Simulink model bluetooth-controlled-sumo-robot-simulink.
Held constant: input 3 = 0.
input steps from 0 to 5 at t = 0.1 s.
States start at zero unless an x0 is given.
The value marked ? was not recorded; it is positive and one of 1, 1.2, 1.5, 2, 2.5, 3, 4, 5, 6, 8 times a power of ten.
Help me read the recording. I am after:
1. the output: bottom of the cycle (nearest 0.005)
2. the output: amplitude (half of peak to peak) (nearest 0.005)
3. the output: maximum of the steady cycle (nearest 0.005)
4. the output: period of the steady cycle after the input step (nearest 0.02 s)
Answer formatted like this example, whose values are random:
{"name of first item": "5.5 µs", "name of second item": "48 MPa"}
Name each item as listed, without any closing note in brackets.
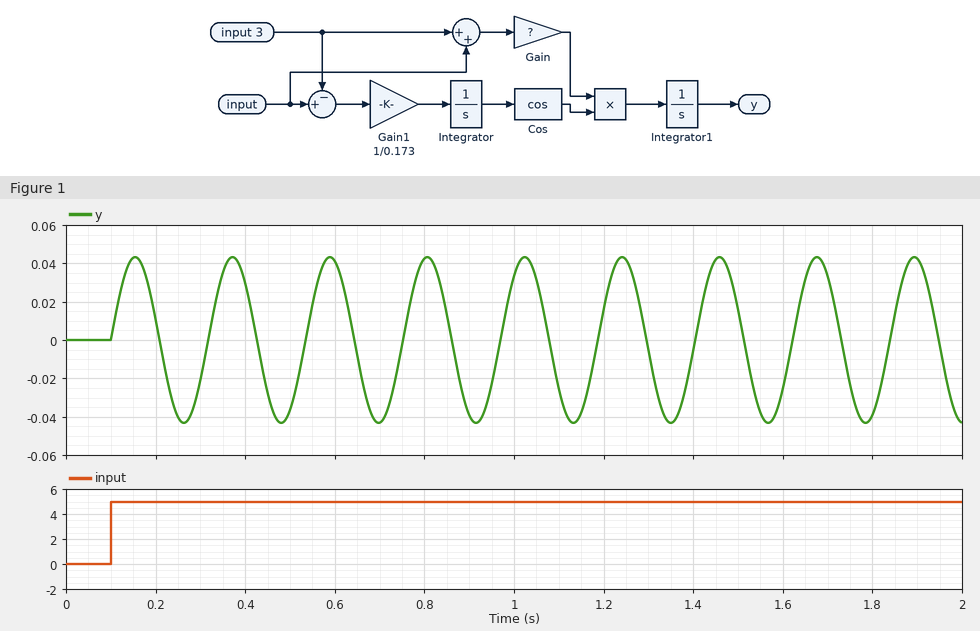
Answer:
{"the output: bottom of the cycle": "-0.045", "the output: amplitude (half of peak to peak)": "0.045", "the output: maximum of the steady cycle": "0.045", "the output: period of the steady cycle after the input step": "0.22 s"}
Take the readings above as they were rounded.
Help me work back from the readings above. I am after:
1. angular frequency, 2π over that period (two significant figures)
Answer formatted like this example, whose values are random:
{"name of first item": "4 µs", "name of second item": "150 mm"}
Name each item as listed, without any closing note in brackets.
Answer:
{"angular frequency, 2π over that period": "29 rad/s"}
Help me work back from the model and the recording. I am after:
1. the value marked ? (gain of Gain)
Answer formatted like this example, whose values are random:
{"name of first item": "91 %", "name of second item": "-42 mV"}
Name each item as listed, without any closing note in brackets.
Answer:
{"the value marked ?": "0.25"}
